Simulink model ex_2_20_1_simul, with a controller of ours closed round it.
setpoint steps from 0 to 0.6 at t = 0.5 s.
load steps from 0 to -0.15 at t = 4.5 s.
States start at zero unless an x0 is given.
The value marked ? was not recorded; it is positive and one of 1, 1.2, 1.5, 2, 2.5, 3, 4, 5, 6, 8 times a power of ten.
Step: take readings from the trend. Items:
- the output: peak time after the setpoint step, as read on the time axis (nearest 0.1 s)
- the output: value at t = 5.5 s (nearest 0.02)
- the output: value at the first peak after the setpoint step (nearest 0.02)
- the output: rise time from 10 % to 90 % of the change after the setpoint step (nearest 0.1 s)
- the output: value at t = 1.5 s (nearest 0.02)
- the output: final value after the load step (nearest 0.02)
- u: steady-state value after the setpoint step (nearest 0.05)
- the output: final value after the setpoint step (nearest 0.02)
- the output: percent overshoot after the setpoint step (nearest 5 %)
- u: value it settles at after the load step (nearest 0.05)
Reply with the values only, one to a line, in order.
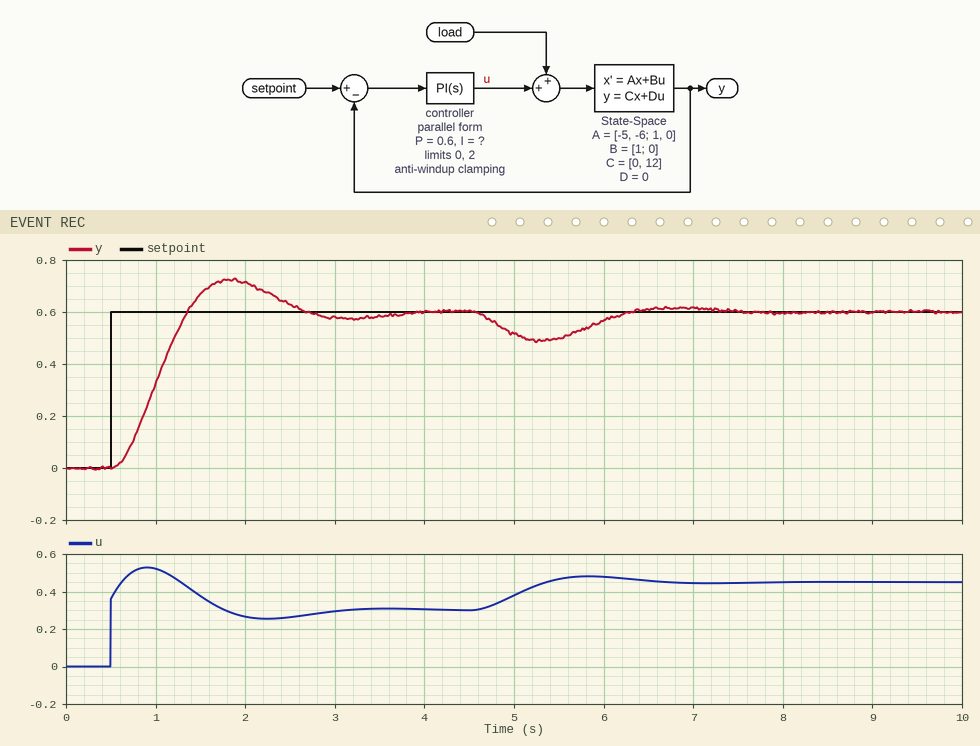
1.8 s
0.50
0.72
0.6 s
0.66
0.60
0.30
0.60
20 %
0.45
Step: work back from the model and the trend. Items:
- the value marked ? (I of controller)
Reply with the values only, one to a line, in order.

1.5
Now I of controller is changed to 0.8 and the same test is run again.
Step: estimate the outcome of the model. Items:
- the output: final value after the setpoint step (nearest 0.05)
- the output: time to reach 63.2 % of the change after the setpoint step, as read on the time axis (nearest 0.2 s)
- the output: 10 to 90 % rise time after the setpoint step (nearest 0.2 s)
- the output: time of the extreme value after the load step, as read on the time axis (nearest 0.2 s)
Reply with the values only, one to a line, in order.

0.60
1.2 s
0.8 s
5.4 s
